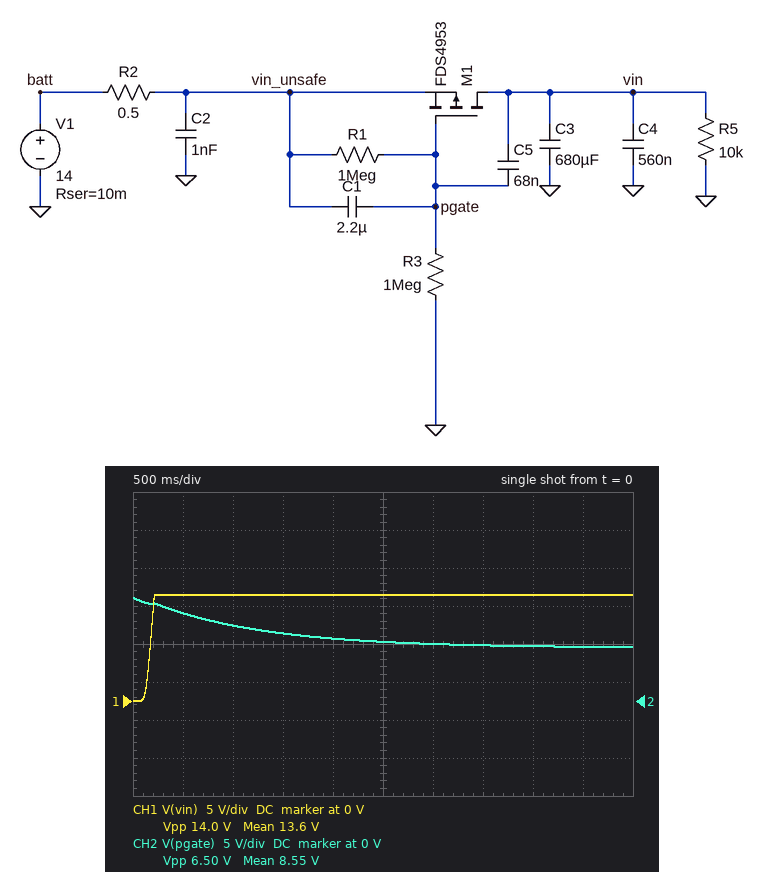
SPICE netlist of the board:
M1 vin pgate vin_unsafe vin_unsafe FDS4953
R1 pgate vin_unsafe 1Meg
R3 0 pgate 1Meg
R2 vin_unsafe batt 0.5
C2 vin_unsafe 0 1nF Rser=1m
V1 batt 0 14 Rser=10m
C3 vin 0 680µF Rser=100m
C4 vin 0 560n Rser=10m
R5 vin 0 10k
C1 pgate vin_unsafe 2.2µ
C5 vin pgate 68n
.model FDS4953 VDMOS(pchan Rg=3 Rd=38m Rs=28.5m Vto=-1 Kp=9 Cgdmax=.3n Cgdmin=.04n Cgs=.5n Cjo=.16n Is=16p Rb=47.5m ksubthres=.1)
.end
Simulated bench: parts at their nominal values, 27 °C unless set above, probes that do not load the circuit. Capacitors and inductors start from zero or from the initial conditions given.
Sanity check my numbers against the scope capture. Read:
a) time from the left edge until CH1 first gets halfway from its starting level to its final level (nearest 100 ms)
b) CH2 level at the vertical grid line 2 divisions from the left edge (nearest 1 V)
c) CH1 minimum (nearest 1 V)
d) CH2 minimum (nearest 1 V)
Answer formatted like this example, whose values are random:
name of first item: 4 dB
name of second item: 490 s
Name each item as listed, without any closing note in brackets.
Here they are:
time from the left edge until CH1 first gets halfway from its starting level to its final level: 200 ms
CH2 level at the vertical grid line 2 divisions from the left edge: 10 V
CH1 minimum: 0 V
CH2 minimum: 7 V
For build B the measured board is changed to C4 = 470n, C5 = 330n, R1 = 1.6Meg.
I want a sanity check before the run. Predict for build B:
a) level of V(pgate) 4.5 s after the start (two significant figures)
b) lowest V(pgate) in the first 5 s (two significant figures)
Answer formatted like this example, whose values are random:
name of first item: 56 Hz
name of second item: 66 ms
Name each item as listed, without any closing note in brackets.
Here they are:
level of V(pgate) 4.5 s after the start: 5.9 V
lowest V(pgate) in the first 5 s: 5.7 V
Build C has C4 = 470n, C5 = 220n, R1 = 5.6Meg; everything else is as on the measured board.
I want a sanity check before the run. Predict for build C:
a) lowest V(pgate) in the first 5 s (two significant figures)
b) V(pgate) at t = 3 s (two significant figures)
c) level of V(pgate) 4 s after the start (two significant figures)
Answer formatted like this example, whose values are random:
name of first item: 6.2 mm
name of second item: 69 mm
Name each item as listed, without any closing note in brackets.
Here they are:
lowest V(pgate) in the first 5 s: 3.2 V
V(pgate) at t = 3 s: 4.9 V
level of V(pgate) 4 s after the start: 3.8 V
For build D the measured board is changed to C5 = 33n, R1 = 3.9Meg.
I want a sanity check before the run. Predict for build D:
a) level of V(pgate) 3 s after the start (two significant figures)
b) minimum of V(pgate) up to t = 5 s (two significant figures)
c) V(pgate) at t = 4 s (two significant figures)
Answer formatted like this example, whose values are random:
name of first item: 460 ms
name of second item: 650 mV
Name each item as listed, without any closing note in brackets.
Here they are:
level of V(pgate) 3 s after the start: 4.9 V
minimum of V(pgate) up to t = 5 s: 3.5 V
V(pgate) at t = 4 s: 4.0 V
